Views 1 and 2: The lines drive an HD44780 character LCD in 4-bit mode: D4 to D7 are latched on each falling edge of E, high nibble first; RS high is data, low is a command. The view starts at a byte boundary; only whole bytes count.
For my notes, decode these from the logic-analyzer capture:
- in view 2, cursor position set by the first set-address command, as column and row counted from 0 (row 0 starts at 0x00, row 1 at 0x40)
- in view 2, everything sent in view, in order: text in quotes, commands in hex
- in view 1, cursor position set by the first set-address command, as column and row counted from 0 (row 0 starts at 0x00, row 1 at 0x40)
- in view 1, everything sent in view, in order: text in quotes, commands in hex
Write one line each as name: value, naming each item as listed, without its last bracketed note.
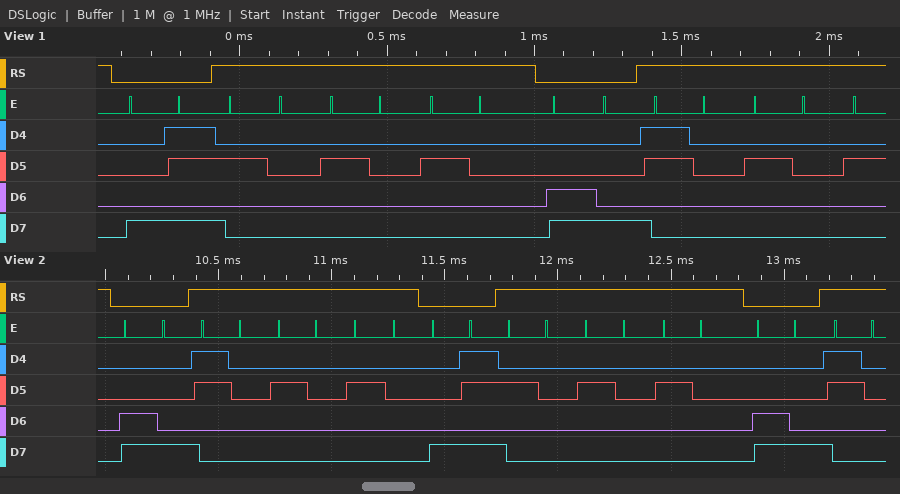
in view 2, cursor position set by the first set-address command, as column and row counted from 0: column 8, row 1
in view 2, everything sent in view, in order: text in quotes, commands in hex: 0xC8 "0  " 0x8B "   " 0xC8 "0"
in view 1, cursor position set by the first set-address command, as column and row counted from 0: column 11, row 0
in view 1, everything sent in view, in order: text in quotes, commands in hex: 0x8B "   " 0xC8 "0 "
